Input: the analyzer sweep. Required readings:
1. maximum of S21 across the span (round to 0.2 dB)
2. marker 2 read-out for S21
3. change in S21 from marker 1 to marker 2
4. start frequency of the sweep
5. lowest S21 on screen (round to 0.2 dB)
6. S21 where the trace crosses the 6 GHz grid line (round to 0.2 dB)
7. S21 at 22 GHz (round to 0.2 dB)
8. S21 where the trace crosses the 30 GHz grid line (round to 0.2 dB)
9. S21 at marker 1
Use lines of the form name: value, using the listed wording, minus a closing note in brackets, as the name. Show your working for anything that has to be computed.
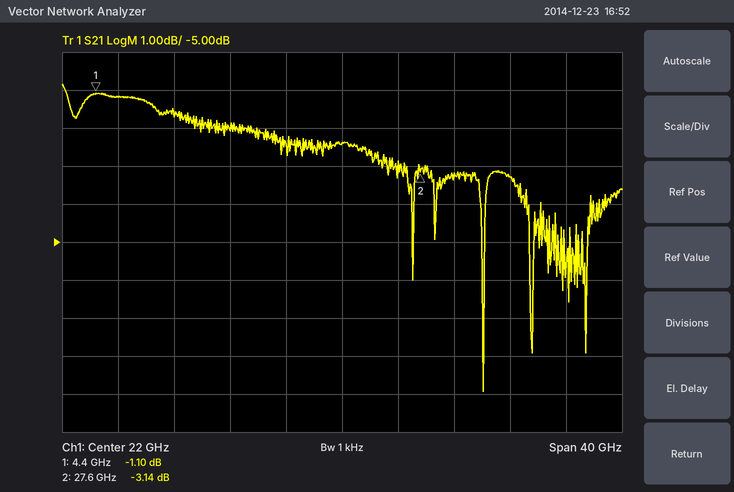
maximum of S21 across the span: -0.8 dB
marker 2 read-out for S21: -3.14 dB
change in S21 from marker 1 to marker 2: -3.14 − (-1.1) = -2.04 dB
start frequency of the sweep: 2 GHz
lowest S21 on screen: -9.0 dB
S21 where the trace crosses the 6 GHz grid line: -1.2 dB
S21 at 22 GHz: -2.4 dB
S21 where the trace crosses the 30 GHz grid line: -3.2 dB
S21 at marker 1: -1.10 dB
